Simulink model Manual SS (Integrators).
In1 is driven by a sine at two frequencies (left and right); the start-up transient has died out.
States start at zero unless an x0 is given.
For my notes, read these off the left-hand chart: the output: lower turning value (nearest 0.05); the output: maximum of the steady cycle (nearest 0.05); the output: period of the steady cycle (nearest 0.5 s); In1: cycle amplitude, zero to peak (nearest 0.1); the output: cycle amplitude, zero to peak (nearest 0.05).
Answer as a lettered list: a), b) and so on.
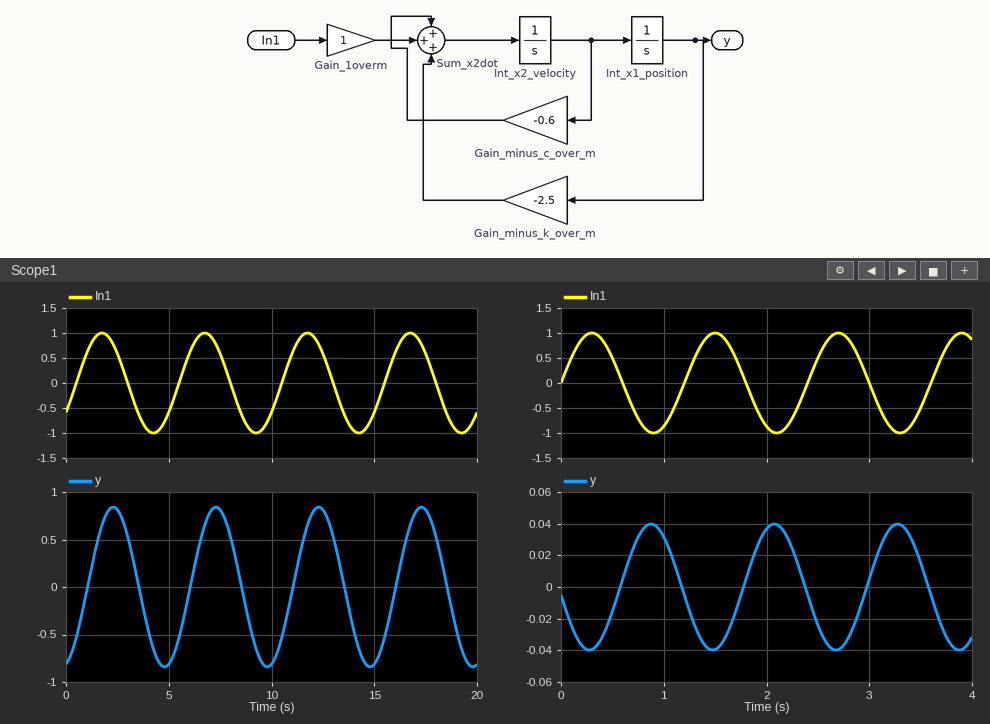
a) -0.85
b) 0.85
c) 5.0 s
d) 1.0
e) 0.85
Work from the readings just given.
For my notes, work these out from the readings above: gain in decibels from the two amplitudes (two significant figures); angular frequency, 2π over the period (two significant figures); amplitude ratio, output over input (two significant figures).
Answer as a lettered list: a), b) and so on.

a) -1.4 dB
b) 1.3 rad/s
c) 0.85
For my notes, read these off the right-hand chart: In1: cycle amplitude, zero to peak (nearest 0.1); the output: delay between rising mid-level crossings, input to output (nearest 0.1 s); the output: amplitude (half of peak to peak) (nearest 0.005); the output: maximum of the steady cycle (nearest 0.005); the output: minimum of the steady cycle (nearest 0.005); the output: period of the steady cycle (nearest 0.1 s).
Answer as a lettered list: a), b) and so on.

a) 1.0
b) 0.6 s
c) 0.040
d) 0.040
e) -0.040
f) 1.2 s
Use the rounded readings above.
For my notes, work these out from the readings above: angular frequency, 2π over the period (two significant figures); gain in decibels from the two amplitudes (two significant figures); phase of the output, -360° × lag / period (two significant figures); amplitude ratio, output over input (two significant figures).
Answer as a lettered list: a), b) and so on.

a) 5.2 rad/s
b) -28 dB
c) -180°
d) 0.040
